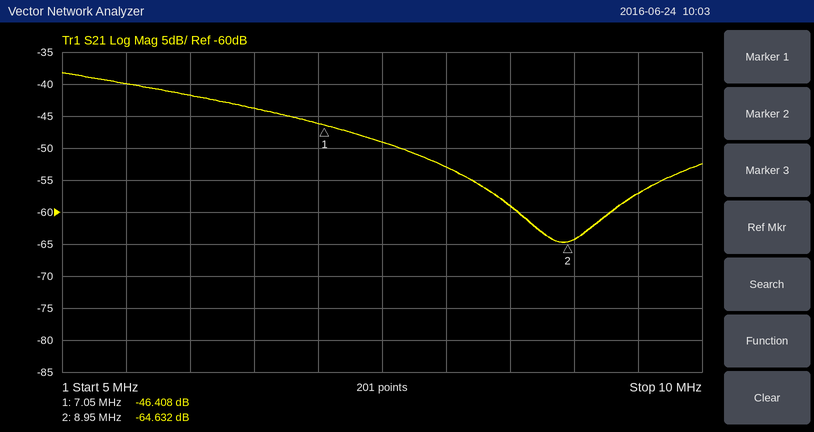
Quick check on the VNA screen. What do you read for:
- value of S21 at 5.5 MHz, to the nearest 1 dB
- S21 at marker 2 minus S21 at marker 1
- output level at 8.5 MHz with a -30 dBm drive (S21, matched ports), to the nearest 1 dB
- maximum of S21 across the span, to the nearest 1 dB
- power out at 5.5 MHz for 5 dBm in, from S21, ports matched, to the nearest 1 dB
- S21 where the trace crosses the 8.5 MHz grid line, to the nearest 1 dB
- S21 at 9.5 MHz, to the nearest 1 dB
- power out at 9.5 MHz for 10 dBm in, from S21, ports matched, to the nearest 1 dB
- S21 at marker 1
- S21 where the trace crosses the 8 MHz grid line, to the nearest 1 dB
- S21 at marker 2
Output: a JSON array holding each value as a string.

["-40 dB", "-18.224 dB", "-89 dBm", "-38 dB", "-35 dBm", "-59 dB", "-57 dB", "-47 dBm", "-46.408 dB", "-53 dB", "-64.632 dB"]
